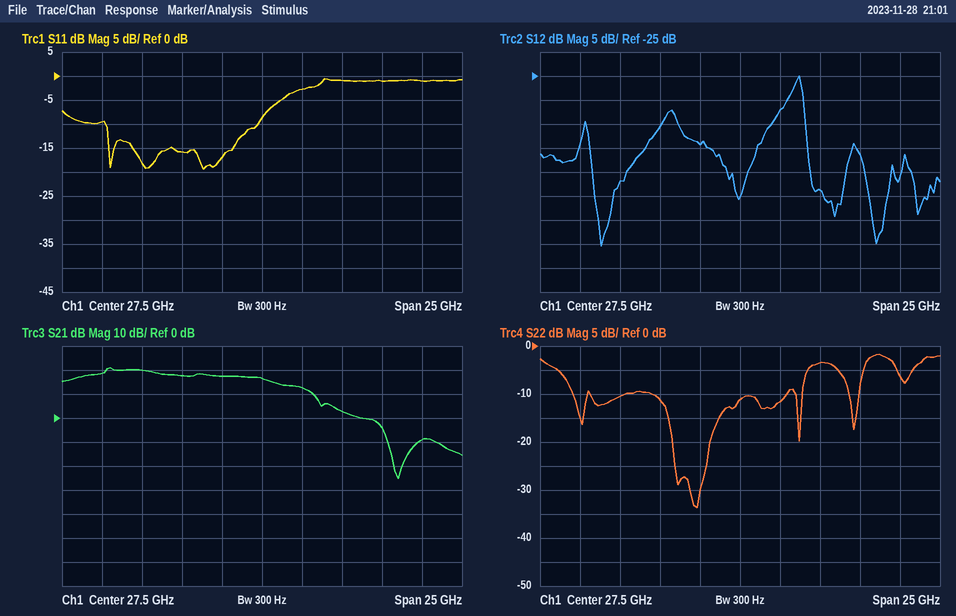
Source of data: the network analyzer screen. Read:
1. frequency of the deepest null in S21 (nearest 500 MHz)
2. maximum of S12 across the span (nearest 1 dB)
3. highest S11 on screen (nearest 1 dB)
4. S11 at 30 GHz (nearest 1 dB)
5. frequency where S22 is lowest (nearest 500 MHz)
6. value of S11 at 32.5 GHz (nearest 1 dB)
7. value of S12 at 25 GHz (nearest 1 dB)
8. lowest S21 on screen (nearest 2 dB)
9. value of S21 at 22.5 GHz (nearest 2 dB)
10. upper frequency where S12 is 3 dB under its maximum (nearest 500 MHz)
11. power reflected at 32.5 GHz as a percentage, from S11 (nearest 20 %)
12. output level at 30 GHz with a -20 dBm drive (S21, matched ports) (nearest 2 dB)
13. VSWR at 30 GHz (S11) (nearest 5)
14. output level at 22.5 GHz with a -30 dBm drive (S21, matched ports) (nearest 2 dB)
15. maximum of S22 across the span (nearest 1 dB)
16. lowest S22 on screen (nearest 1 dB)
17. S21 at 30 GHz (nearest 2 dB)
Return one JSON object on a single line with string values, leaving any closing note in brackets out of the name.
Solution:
{"frequency of the deepest null in S21": "36.0 GHz", "maximum of S12 across the span": "-25 dB", "highest S11 on screen": "-1 dB", "S11 at 30 GHz": "-3 dB", "frequency where S22 is lowest": "25.0 GHz", "value of S11 at 32.5 GHz": "-1 dB", "value of S12 at 25 GHz": "-39 dB", "lowest S21 on screen": "-26 dB", "value of S21 at 22.5 GHz": "18 dB", "upper frequency where S12 is 3 dB under its maximum": "31.5 GHz", "power reflected at 32.5 GHz as a percentage, from S11": "80 %", "output level at 30 GHz with a -20 dBm drive (S21, matched ports)": "-8 dBm", "VSWR at 30 GHz (S11)": "5", "output level at 22.5 GHz with a -30 dBm drive (S21, matched ports)": "-12 dBm", "maximum of S22 across the span": "-2 dB", "lowest S22 on screen": "-34 dB", "S21 at 30 GHz": "12 dB"}
